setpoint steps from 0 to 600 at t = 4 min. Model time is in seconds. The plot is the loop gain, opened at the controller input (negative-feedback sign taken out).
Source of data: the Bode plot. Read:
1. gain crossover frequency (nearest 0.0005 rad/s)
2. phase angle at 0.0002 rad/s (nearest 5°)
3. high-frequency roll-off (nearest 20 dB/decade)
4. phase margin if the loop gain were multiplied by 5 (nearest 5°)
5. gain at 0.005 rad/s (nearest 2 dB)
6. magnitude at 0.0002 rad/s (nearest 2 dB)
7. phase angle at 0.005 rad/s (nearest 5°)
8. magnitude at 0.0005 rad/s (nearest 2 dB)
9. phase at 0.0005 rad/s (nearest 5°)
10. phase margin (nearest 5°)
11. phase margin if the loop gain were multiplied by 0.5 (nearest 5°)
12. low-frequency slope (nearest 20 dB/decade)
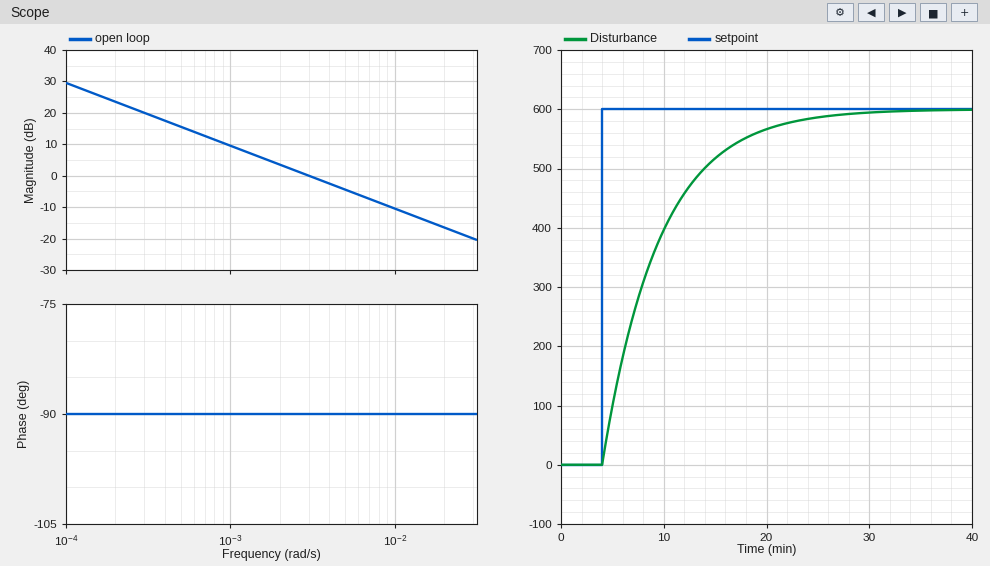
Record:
0.0030 rad/s
-90°
-20 dB/decade
90°
-4 dB
24 dB
-90°
16 dB
-90°
90°
90°
-20 dB/decade
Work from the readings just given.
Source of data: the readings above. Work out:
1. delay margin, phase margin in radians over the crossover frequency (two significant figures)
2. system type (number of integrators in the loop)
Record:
520 s
1
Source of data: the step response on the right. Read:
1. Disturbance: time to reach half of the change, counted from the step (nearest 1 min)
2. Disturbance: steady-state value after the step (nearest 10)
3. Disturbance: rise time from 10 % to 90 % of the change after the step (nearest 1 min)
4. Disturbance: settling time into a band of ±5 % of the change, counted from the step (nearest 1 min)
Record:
4 min
600
12 min
17 min
